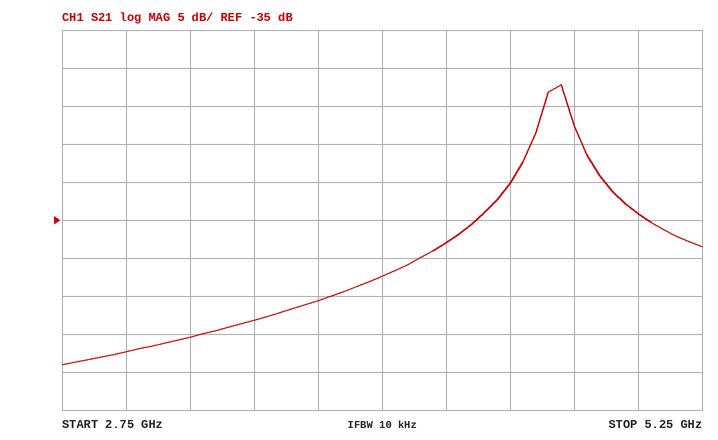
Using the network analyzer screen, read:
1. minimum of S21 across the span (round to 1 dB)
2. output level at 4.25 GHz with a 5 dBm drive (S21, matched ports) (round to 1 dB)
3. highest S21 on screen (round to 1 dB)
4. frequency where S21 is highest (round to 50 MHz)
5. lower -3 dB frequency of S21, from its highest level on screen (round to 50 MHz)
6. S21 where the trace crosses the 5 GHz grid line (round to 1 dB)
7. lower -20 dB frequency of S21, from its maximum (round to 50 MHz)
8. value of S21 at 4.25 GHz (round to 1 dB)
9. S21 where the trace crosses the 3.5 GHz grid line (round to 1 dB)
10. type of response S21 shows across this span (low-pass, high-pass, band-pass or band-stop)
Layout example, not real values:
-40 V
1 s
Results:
-54 dB
-33 dBm
-17 dB
4.70 GHz
4.65 GHz
-34 dB
4.30 GHz
-38 dB
-48 dB
band-pass
